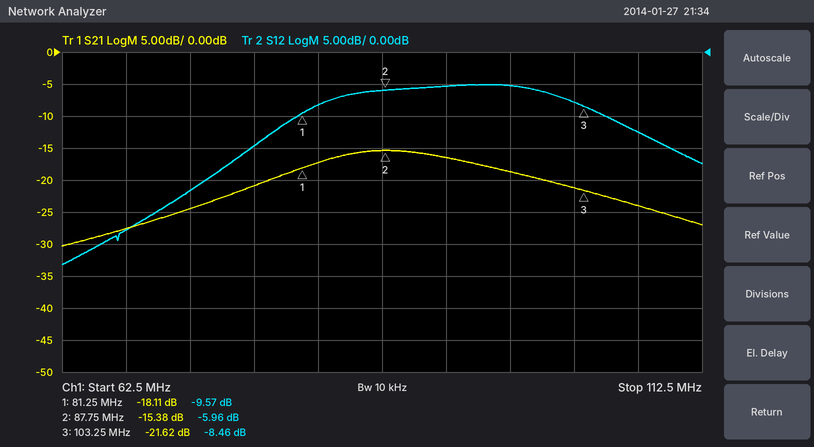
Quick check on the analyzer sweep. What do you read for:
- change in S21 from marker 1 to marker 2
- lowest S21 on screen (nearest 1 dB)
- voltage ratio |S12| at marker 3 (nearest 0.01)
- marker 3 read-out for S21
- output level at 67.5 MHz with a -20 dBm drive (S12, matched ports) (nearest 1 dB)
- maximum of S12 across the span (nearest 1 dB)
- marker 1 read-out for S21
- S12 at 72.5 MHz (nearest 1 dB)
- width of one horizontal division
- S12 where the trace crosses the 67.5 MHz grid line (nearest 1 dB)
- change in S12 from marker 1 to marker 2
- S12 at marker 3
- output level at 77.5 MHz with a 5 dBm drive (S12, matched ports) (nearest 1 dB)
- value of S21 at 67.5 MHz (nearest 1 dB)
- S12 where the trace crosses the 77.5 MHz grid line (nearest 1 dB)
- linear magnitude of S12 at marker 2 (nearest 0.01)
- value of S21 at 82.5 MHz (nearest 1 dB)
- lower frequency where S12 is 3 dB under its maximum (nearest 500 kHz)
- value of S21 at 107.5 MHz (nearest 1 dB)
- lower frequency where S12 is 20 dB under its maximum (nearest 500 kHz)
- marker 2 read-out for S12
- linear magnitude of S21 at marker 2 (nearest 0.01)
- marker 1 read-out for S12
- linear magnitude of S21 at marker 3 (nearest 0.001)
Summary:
2.73 dB
-30 dB
0.38
-21.62 dB
-48 dBm
-5 dB
-18.11 dB
-22 dB
5 MHz
-28 dB
3.61 dB
-8.46 dB
-10 dBm
-28 dB
-15 dB
0.50
-17 dB
82.5 MHz
-24 dB
70.0 MHz
-5.96 dB
0.17
-9.57 dB
0.083
